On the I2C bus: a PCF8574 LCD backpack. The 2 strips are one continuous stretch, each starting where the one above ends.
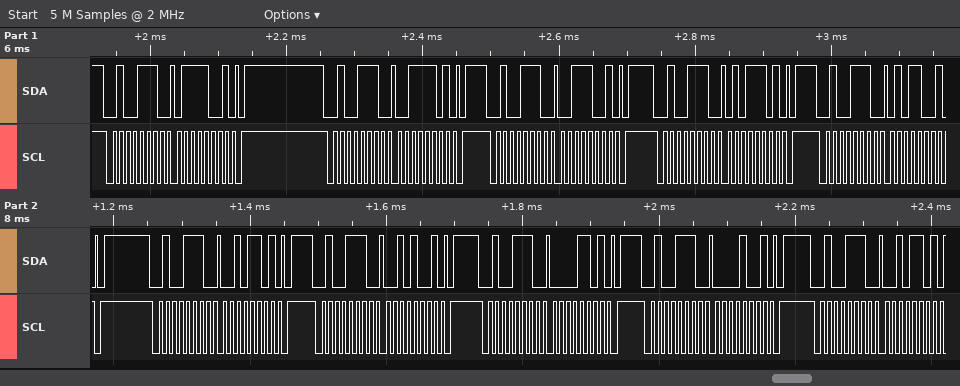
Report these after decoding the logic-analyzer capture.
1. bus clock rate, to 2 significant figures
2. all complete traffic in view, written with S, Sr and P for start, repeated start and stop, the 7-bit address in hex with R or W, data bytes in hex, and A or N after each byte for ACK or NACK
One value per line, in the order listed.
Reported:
100 kHz
S 27W A 79 A P S 27W A 3D A P S 27W A 39 A P S 27W A 5D A P S 27W A 59 A P S 27W A 2D A P S 27W A 29 A P S 27W A 0D A P S 27W A 09 A P S 27W A 2D A
